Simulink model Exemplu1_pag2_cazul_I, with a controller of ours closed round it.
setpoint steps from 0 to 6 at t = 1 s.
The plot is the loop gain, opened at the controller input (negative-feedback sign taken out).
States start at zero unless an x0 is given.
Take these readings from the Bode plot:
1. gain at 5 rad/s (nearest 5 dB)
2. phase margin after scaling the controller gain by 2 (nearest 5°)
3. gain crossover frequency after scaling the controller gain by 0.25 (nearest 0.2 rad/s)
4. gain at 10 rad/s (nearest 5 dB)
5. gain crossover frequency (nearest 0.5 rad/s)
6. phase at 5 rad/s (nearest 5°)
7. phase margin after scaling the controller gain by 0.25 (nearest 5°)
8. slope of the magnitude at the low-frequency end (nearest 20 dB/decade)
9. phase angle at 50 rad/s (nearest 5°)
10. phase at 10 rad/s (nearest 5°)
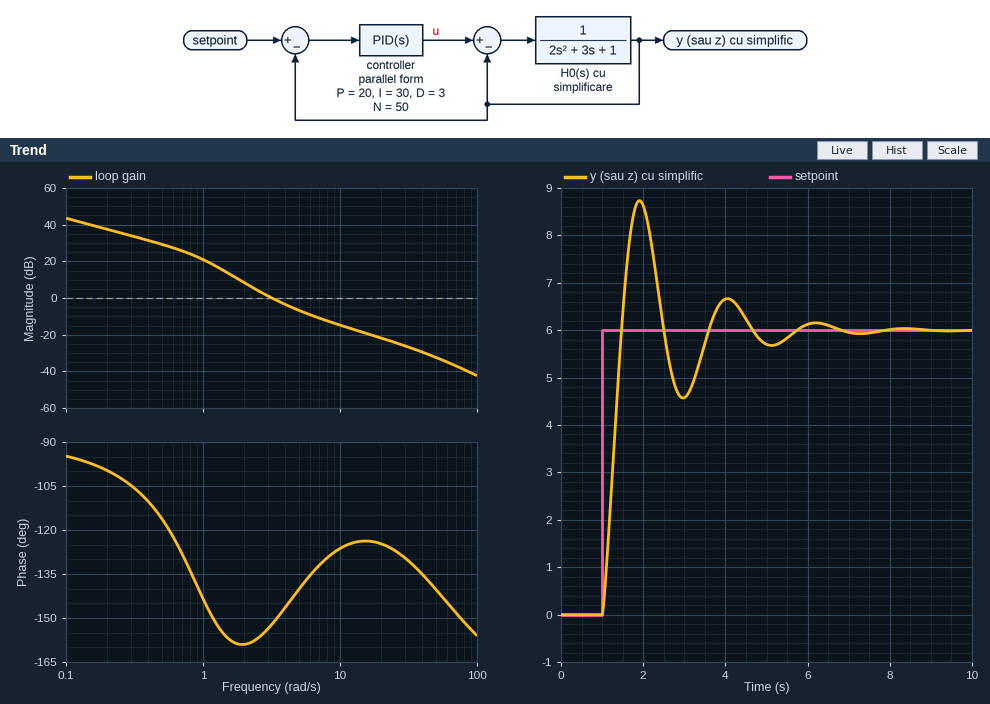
-5 dB
40°
1.6 rad/s
-15 dB
3.0 rad/s
-140°
20°
-20 dB/decade
-140°
-125°
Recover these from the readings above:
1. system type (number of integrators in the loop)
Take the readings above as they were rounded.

1
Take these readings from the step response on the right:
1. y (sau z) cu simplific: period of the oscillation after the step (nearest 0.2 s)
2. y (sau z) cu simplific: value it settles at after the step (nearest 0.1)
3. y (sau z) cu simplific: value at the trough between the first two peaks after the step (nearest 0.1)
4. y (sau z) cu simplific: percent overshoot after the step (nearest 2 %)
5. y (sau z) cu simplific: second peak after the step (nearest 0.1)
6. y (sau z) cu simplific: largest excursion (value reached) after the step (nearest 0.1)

2.2 s
6.0
4.6
46 %
6.7
8.7
